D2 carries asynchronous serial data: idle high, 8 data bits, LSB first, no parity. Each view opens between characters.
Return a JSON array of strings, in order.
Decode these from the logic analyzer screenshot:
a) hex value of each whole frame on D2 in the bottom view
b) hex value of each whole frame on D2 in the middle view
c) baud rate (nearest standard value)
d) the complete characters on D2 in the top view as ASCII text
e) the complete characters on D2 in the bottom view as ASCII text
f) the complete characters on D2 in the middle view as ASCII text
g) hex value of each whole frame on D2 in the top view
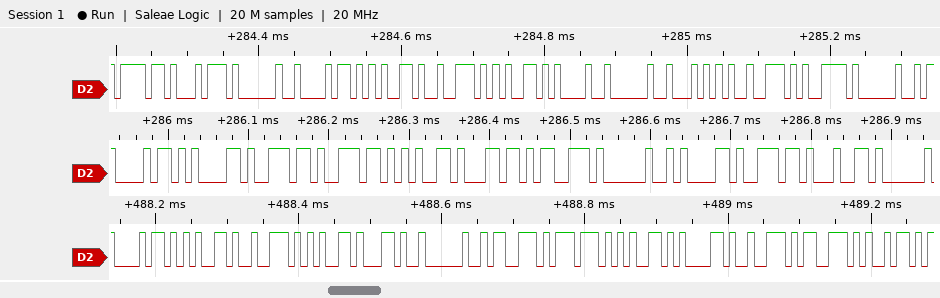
["68, 65, 72, 65, 2C, 20, 73, 77, 65, 61, 72, 73, 69", "68, 61, 6E, 6E, 65, 6C, 73, 20, 61, 6E, 64", "115200 baud", "\"ot here! Try \"", "\"here, swearsi\"", "\"hannels and\"", "6F, 74, 20, 68, 65, 72, 65, 21, 20, 54, 72, 79, 20"]
